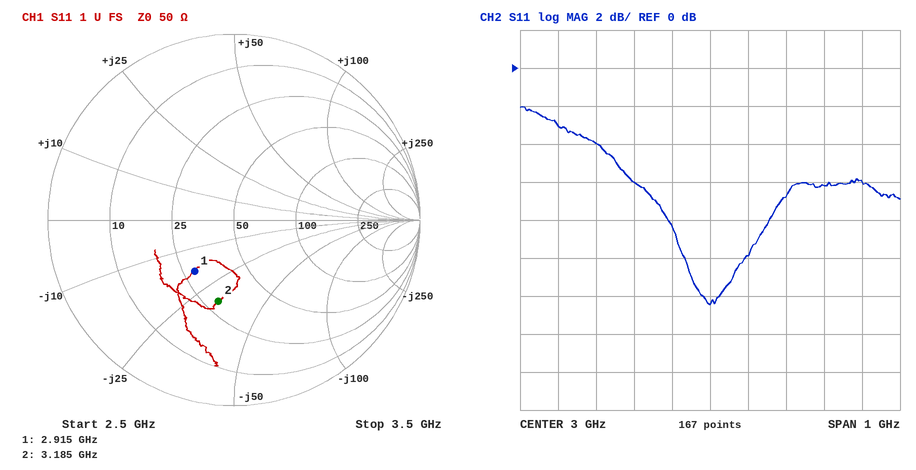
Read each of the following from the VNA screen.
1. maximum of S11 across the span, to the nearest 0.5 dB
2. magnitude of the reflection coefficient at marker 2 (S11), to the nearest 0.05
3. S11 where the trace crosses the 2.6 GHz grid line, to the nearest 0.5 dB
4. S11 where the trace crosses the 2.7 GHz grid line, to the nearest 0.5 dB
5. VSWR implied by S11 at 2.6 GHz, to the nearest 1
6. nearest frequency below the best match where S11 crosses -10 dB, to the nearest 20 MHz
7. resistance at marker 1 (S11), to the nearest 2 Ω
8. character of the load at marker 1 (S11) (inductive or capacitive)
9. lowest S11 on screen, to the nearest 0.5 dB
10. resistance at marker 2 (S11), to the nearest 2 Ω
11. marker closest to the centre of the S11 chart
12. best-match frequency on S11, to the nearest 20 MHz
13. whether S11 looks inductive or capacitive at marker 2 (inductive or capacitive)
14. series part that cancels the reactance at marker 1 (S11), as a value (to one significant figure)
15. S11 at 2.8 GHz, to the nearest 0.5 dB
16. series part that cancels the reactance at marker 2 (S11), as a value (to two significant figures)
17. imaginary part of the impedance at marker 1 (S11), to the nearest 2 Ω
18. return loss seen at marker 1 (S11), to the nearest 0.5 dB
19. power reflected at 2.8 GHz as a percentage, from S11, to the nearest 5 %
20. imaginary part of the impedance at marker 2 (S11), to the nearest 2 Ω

-2.0 dB
0.45
-3.0 dB
-4.0 dB
6
2.94 GHz
28 Ω
capacitive
-12.5 dB
30 Ω
marker 1
3.00 GHz
capacitive
1.0 nH
-6.0 dB
1.6 nH
-18 Ω
9.0 dB
25 %
-32 Ω
